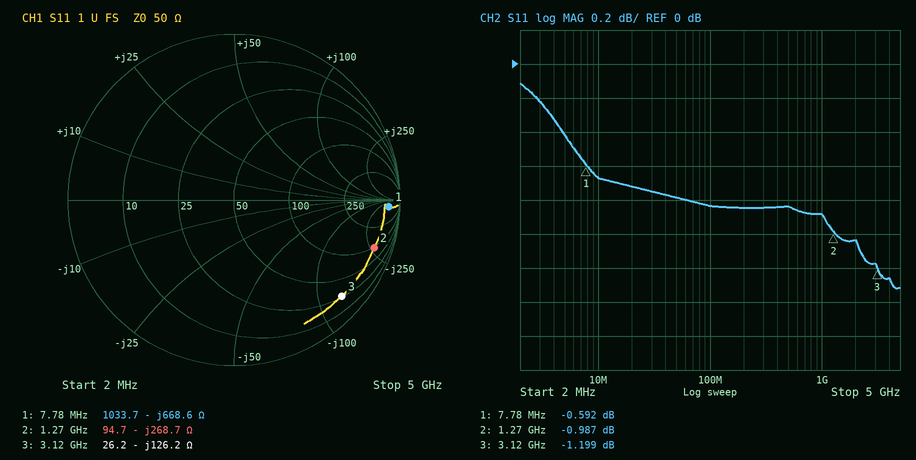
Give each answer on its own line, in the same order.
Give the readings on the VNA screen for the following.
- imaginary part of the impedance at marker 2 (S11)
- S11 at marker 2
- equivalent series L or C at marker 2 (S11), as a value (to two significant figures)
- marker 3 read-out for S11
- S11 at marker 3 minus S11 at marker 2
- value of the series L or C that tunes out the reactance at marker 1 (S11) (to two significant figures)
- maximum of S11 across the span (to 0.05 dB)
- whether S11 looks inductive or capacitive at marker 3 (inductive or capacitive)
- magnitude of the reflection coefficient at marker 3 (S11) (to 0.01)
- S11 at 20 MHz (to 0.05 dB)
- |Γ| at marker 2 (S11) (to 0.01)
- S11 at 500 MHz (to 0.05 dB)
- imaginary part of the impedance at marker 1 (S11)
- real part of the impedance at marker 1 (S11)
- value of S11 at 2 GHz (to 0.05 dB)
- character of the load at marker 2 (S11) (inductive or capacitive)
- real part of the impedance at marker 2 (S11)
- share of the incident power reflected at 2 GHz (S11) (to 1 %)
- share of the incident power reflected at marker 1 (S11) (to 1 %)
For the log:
-268.7 Ω
-0.987 dB
470 fF
-1.199 dB
-0.212 dB
14 µH
-0.10 dB
capacitive
0.87
-0.70 dB
0.89
-0.85 dB
-668.6 Ω
1033.7 Ω
-1.05 dB
capacitive
94.7 Ω
79 %
87 %
